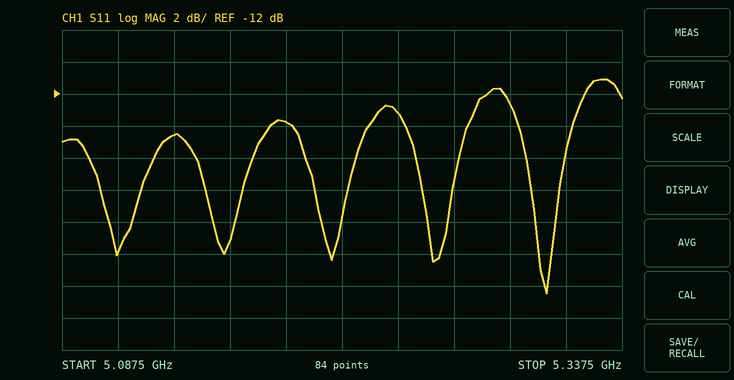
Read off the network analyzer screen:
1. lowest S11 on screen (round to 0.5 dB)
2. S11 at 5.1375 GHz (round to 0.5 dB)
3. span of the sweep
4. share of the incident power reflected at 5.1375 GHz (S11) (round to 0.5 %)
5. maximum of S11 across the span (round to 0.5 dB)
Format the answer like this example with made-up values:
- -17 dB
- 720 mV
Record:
- -24.5 dB
- -14.5 dB
- 250 MHz
- 3.5 %
- -11.0 dB
